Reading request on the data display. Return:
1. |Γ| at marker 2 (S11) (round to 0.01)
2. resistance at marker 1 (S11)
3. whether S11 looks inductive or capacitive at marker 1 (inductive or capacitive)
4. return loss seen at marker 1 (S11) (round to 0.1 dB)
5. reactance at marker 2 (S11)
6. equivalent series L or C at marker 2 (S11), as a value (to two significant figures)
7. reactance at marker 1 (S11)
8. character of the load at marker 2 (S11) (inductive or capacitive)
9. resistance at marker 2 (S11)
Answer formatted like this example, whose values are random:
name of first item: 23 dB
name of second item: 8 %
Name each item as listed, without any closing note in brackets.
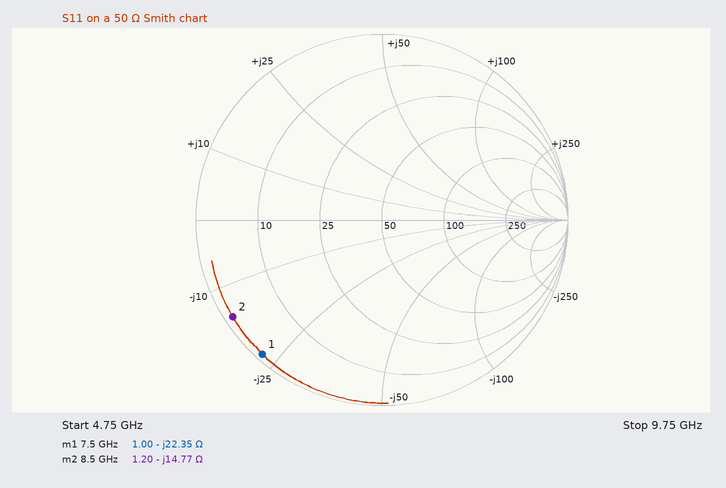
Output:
|Γ| at marker 2 (S11): 0.96
resistance at marker 1: 1.00 Ω
whether S11 looks inductive or capacitive at marker 1: capacitive
return loss seen at marker 1 (S11): 0.3 dB
reactance at marker 2: -14.77 Ω
equivalent series L or C at marker 2 (S11), as a value: 1.3 pF
reactance at marker 1: -22.35 Ω
character of the load at marker 2 (S11): capacitive
resistance at marker 2: 1.20 Ω
